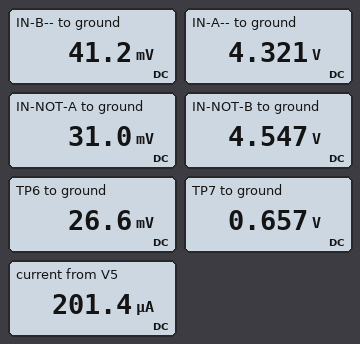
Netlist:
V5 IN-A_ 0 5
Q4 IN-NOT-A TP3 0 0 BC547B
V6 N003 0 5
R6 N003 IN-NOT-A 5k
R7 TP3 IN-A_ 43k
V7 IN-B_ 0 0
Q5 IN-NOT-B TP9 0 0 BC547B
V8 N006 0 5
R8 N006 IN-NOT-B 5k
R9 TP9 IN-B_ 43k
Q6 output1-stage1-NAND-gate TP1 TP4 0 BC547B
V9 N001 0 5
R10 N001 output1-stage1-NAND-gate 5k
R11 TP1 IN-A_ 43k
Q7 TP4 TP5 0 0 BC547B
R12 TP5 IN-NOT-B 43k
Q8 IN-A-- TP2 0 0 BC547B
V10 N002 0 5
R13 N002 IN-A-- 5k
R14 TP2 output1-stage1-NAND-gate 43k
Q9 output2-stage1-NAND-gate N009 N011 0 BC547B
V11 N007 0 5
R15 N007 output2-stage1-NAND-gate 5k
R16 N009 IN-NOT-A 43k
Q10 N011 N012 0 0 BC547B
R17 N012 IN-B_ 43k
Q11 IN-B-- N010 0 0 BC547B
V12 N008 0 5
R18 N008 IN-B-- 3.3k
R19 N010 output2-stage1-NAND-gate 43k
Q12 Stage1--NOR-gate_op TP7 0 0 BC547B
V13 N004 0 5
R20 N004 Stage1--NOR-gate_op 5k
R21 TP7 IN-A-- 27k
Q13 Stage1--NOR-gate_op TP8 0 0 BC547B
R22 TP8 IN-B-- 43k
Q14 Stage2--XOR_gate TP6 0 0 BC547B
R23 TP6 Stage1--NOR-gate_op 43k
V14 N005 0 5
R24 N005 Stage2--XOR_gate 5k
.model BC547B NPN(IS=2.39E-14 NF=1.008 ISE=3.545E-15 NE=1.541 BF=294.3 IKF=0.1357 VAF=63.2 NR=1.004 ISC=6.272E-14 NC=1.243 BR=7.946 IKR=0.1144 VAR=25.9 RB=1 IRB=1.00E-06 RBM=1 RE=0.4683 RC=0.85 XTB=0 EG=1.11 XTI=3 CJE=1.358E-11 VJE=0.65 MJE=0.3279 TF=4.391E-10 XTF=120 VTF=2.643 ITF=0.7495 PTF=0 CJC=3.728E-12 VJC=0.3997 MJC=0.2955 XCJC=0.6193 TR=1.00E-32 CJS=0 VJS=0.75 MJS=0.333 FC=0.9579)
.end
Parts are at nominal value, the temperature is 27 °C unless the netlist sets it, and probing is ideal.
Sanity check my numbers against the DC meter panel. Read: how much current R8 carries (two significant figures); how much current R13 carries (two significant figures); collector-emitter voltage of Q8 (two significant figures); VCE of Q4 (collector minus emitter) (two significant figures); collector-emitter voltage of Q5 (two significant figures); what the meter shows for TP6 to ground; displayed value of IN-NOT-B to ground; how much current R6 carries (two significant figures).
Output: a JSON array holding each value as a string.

["91 µA", "140 µA", "4.3 V", "31 mV", "4.5 V", "26.6 mV", "4.547 V", "990 µA"]
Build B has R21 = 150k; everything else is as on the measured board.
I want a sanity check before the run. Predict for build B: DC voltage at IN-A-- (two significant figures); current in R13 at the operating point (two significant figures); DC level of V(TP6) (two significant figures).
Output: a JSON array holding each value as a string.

["4.9 V", "28 µA", "58 mV"]
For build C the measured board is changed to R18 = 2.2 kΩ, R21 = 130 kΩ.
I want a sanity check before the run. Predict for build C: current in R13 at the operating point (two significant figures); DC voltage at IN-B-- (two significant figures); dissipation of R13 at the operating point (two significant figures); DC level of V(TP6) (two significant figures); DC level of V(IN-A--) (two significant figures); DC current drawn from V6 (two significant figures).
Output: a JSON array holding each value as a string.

["32 µA", "51 mV", "5.2 µW", "55 mV", "4.8 V", "990 µA"]
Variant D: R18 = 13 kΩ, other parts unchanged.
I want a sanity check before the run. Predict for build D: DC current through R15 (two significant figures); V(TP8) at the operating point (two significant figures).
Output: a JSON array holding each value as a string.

["91 µA", "19 mV"]
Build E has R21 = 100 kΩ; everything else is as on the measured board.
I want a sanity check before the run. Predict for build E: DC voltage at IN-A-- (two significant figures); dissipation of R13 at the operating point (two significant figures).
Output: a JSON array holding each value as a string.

["4.8 V", "8.6 µW"]
